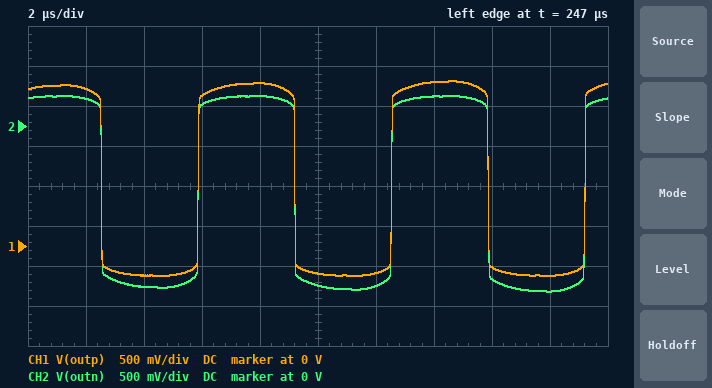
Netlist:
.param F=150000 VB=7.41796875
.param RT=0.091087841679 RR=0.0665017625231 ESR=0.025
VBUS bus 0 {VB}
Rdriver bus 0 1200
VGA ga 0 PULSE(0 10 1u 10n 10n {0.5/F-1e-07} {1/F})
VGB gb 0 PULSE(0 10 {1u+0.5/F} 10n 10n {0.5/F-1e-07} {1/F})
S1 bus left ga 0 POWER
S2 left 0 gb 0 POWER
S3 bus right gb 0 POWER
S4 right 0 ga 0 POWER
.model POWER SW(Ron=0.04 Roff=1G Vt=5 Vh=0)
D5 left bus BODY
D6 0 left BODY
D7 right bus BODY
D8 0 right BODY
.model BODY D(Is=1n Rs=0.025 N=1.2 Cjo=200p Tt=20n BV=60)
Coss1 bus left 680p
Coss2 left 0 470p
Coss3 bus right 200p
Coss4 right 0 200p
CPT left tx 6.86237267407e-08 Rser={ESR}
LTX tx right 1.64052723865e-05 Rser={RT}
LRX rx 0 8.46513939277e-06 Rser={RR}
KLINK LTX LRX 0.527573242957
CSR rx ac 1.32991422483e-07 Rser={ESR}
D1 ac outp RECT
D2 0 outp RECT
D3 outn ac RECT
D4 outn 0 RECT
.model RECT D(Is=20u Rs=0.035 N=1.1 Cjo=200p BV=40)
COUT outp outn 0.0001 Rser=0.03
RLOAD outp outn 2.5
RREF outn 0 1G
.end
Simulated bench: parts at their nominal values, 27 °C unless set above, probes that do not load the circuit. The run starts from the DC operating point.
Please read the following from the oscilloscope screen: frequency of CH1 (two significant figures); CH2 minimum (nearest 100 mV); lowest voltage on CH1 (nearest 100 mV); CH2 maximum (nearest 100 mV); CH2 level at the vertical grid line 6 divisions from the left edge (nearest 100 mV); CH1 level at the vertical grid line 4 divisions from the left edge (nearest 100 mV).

150 kHz
-2.1 V
-400 mV
400 mV
-2.0 V
2.0 V
